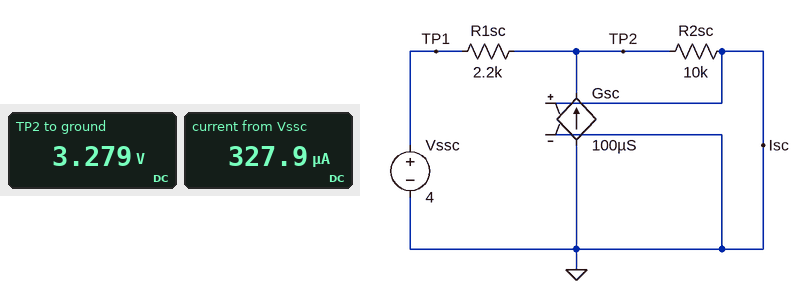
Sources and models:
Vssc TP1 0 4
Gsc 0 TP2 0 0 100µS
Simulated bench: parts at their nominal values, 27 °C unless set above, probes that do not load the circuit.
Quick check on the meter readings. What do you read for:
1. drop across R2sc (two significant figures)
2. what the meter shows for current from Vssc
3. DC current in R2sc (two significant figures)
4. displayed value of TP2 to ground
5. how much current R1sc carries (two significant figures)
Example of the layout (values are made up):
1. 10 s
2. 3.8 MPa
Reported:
1. 3.3 V
2. 327.9 µA
3. 330 µA
4. 3.279 V
5. 330 µA
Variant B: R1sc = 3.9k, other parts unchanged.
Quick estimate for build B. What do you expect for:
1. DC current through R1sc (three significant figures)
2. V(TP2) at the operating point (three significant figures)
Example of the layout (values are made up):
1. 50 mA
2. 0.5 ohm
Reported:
1. 288 µA
2. 2.88 V
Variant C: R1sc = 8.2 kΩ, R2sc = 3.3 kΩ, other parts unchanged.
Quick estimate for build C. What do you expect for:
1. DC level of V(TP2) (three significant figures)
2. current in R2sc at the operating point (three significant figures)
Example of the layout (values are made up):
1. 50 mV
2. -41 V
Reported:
1. 1.15 V
2. 348 µA
